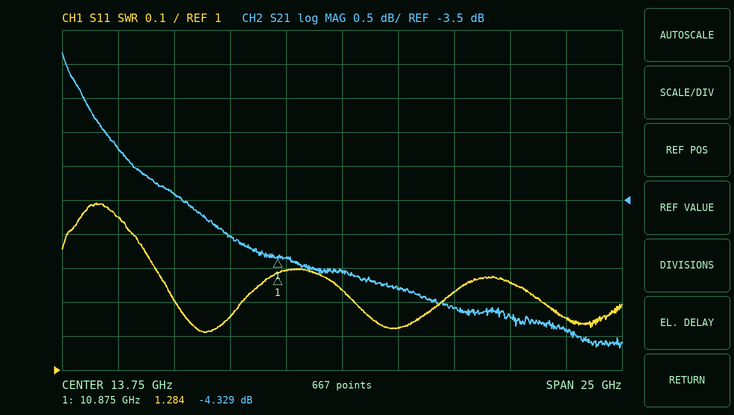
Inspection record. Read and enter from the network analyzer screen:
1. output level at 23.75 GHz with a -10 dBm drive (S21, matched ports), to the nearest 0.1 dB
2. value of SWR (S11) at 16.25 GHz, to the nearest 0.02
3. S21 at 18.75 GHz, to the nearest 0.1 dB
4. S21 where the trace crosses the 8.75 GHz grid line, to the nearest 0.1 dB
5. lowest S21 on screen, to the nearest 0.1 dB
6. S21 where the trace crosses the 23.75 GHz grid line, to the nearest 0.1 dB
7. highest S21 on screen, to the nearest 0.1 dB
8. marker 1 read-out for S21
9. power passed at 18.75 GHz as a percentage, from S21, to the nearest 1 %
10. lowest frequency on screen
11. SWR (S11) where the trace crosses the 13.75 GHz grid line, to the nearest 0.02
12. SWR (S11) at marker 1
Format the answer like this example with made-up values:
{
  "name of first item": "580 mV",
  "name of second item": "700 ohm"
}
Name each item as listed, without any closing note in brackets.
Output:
{
  "output level at 23.75 GHz with a -10 dBm drive (S21, matched ports), to the nearest 0.1 dB": "-15.4 dBm",
  "value of SWR (S11) at 16.25 GHz, to the nearest 0.02": "1.12",
  "S21 at 18.75 GHz, to the nearest 0.1 dB": "-5.1 dB",
  "S21 where the trace crosses the 8.75 GHz grid line, to the nearest 0.1 dB": "-4.0 dB",
  "lowest S21 on screen, to the nearest 0.1 dB": "-5.7 dB",
  "S21 where the trace crosses the 23.75 GHz grid line, to the nearest 0.1 dB": "-5.4 dB",
  "highest S21 on screen, to the nearest 0.1 dB": "-1.3 dB",
  "marker 1 read-out for S21": "-4.329 dB",
  "power passed at 18.75 GHz as a percentage, from S21, to the nearest 1 %": "31 %",
  "lowest frequency on screen": "1.25 GHz",
  "SWR (S11) where the trace crosses the 13.75 GHz grid line, to the nearest 0.02": "1.24",
  "SWR (S11) at marker 1": "1.284"
}
